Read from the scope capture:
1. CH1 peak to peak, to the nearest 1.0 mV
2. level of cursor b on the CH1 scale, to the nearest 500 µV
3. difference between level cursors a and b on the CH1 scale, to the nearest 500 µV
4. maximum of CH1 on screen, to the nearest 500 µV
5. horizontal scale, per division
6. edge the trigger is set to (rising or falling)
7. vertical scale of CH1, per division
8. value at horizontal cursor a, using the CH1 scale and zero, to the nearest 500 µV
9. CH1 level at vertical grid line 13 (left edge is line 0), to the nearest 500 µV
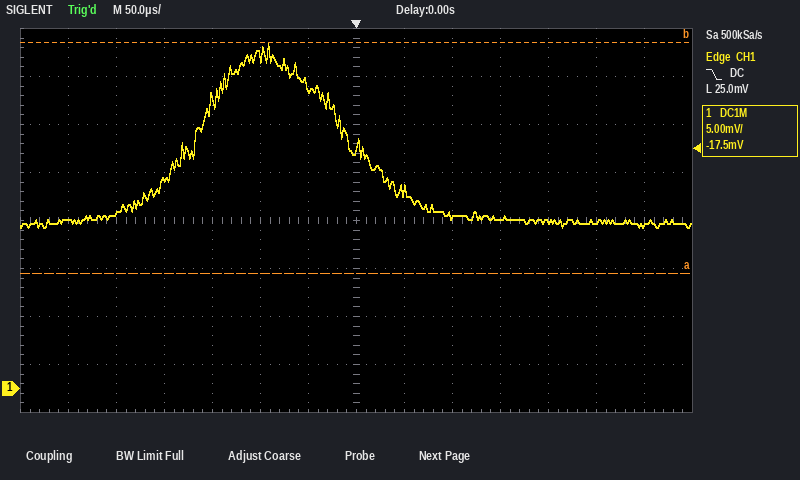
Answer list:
19.0 mV
36.0 mV
24.0 mV
36.0 mV
50 µs
falling
5 mV
12.0 mV
17.0 mV
